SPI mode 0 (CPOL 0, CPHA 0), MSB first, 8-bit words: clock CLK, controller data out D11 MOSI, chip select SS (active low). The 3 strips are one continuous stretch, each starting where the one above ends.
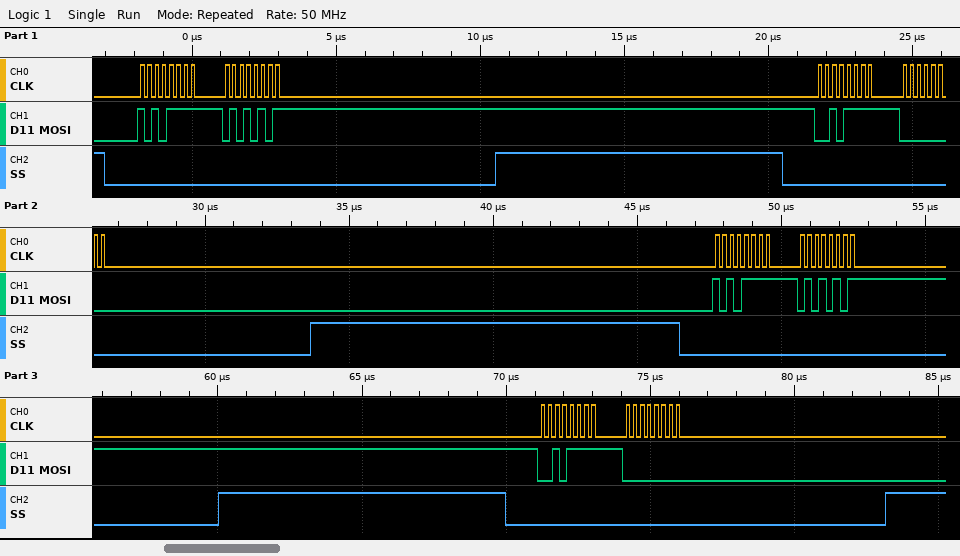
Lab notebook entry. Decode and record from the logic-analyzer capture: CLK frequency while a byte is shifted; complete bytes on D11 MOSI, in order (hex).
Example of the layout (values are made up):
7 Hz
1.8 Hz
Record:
4 MHz
AF 55 2F 00 AF 55 2F 00
